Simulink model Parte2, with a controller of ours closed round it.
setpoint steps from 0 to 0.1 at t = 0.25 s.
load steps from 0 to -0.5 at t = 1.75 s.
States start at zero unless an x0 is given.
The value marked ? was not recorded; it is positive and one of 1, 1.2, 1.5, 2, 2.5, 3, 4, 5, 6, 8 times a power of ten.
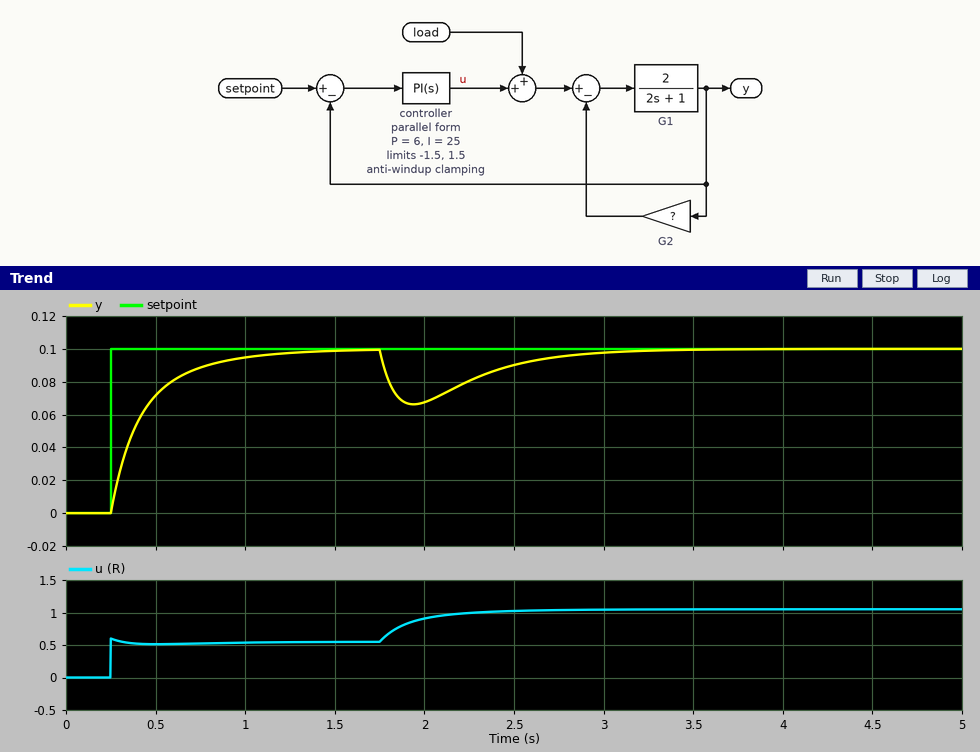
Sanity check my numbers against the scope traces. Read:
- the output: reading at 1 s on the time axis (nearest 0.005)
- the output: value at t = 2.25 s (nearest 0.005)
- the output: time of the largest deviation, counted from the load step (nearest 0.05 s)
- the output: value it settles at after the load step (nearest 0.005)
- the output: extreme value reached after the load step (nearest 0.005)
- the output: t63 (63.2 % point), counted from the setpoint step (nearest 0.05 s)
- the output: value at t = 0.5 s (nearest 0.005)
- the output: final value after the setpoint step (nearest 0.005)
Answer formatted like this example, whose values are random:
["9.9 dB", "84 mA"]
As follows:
["0.095", "0.080", "0.20 s", "0.100", "0.065", "0.20 s", "0.070", "0.100"]
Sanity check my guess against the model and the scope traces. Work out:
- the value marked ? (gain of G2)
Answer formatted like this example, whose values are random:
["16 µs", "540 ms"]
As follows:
["5"]
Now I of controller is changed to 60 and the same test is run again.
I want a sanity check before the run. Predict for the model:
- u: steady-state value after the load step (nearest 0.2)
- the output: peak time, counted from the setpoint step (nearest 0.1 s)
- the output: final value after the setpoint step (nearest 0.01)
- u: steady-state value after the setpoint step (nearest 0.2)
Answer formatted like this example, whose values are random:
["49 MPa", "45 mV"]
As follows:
["1.0", "0.4 s", "0.10", "0.6"]
